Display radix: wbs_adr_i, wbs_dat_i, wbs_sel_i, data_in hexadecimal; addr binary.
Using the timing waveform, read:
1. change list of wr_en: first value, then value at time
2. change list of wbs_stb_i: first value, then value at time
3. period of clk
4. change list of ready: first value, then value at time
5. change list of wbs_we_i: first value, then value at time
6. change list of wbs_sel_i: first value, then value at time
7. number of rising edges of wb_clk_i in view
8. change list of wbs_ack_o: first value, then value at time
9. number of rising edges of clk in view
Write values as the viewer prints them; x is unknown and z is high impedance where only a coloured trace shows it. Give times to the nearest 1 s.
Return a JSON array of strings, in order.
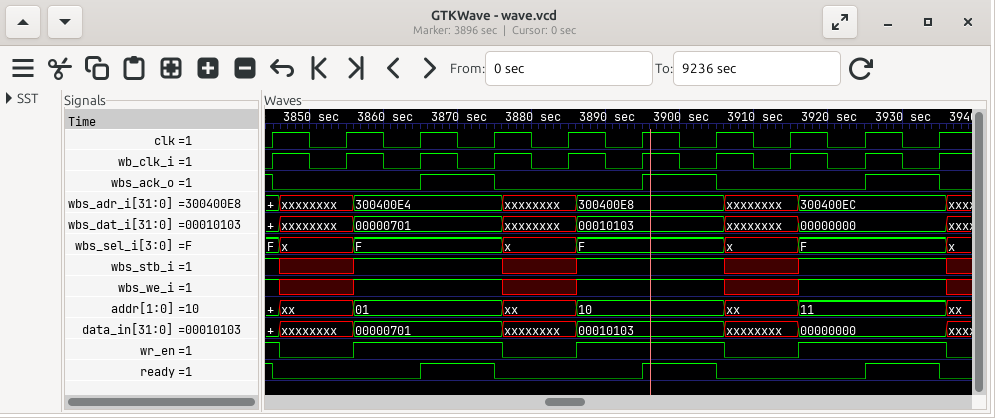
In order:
["1, 0 at 3846 s, 1 at 3856 s, 0 at 3876 s, 1 at 3886 s, 0 at 3906 s, 1 at 3916 s, 0 at 3936 s", "1, x at 3846 s, 1 at 3856 s, x at 3876 s, 1 at 3886 s, x at 3906 s, 1 at 3916 s, x at 3936 s", "10 s", "1, 0 at 3845 s, 1 at 3865 s, 0 at 3875 s, 1 at 3895 s, 0 at 3905 s, 1 at 3925 s, 0 at 3935 s", "1, x at 3846 s, 1 at 3856 s, x at 3876 s, 1 at 3886 s, x at 3906 s, 1 at 3916 s, x at 3936 s", "F, x at 3846 s, F at 3856 s, x at 3876 s, F at 3886 s, x at 3906 s, F at 3916 s, x at 3936 s", "10", "1, 0 at 3845 s, 1 at 3865 s, 0 at 3875 s, 1 at 3895 s, 0 at 3905 s, 1 at 3925 s, 0 at 3935 s", "10"]
